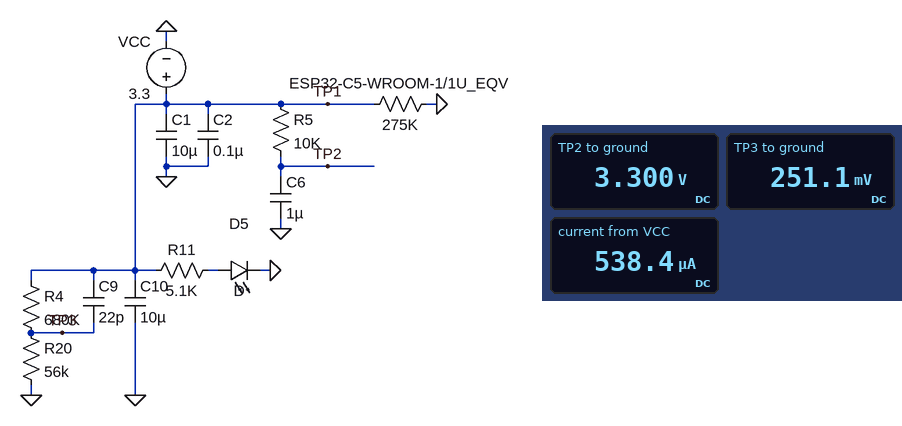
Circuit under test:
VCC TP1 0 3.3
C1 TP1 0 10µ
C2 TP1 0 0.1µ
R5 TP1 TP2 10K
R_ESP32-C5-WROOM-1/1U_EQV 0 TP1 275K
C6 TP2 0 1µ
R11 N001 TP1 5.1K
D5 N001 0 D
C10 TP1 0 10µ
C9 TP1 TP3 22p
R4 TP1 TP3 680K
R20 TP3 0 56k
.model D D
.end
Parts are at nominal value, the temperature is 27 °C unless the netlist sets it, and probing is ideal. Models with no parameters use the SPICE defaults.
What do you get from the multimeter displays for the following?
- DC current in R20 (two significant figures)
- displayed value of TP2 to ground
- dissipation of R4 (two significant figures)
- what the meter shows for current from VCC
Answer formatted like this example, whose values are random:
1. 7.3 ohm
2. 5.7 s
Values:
1. 4.5 µA
2. 3.300 V
3. 14 µW
4. 538.4 µA
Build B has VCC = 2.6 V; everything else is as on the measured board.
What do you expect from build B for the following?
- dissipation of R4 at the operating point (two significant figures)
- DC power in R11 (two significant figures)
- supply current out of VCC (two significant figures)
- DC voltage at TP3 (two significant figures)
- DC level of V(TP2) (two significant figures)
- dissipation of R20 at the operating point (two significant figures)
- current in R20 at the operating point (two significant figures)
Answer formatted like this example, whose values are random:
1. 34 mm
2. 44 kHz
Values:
1. 8.5 µW
2. 760 µW
3. 400 µA
4. 200 mV
5. 2.6 V
6. 700 nW
7. 3.5 µA
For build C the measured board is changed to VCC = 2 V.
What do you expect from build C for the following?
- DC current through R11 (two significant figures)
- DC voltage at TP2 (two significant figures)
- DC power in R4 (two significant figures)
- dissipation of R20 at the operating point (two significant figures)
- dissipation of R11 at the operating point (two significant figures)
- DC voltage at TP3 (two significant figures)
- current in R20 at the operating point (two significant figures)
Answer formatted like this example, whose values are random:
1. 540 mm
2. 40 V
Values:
1. 270 µA
2. 2.0 V
3. 5.0 µW
4. 410 nW
5. 370 µW
6. 150 mV
7. 2.7 µA
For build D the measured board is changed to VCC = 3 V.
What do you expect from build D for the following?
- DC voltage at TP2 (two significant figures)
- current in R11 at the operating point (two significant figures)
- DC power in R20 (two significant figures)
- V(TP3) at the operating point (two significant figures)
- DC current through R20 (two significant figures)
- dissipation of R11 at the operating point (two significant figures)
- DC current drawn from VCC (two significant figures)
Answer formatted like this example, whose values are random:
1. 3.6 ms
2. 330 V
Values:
1. 3.0 V
2. 460 µA
3. 930 nW
4. 230 mV
5. 4.1 µA
6. 1.1 mW
7. 480 µA
